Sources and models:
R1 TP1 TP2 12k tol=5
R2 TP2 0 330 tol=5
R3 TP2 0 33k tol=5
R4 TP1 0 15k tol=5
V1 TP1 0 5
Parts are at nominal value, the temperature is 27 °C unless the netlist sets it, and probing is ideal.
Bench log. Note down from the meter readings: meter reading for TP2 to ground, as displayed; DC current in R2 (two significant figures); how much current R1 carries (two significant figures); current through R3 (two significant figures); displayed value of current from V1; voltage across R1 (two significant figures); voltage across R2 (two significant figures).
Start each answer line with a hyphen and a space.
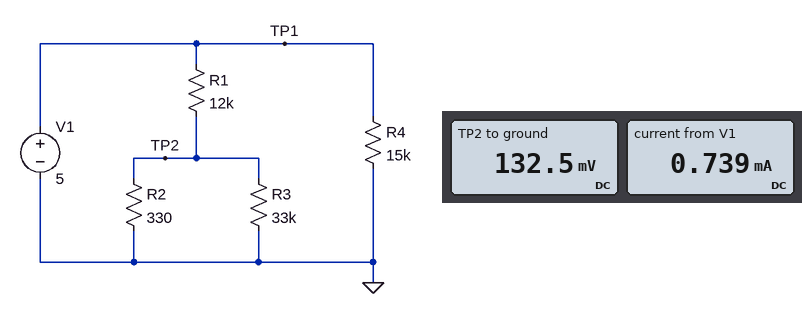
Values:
- 132.5 mV
- 400 µA
- 410 µA
- 4.0 µA
- 0.739 mA
- 4.9 V
- 130 mV
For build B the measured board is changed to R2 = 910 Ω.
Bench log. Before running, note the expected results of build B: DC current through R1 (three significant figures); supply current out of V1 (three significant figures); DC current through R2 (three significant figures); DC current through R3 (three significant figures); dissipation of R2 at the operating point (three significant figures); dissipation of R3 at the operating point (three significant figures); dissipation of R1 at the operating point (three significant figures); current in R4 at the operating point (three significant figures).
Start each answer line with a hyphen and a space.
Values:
- 388 µA
- 721 µA
- 378 µA
- 10.4 µA
- 130 µW
- 3.58 µW
- 1.81 mW
- 333 µA
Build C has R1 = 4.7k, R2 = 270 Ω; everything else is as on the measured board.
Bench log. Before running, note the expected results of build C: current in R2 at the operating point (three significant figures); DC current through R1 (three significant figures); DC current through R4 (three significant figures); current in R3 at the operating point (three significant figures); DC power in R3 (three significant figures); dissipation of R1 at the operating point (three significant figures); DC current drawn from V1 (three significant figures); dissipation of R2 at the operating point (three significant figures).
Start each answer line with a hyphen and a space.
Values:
- 998 µA
- 1.01 mA
- 333 µA
- 8.17 µA
- 2.20 µW
- 4.76 mW
- 1.34 mA
- 269 µW
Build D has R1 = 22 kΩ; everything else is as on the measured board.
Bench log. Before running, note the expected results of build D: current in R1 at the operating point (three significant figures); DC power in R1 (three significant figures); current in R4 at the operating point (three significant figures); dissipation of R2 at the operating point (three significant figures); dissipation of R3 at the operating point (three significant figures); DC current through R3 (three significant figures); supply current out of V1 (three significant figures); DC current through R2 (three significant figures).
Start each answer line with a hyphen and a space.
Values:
- 224 µA
- 1.10 mW
- 333 µA
- 16.2 µW
- 162 nW
- 2.22 µA
- 557 µA
- 222 µA
